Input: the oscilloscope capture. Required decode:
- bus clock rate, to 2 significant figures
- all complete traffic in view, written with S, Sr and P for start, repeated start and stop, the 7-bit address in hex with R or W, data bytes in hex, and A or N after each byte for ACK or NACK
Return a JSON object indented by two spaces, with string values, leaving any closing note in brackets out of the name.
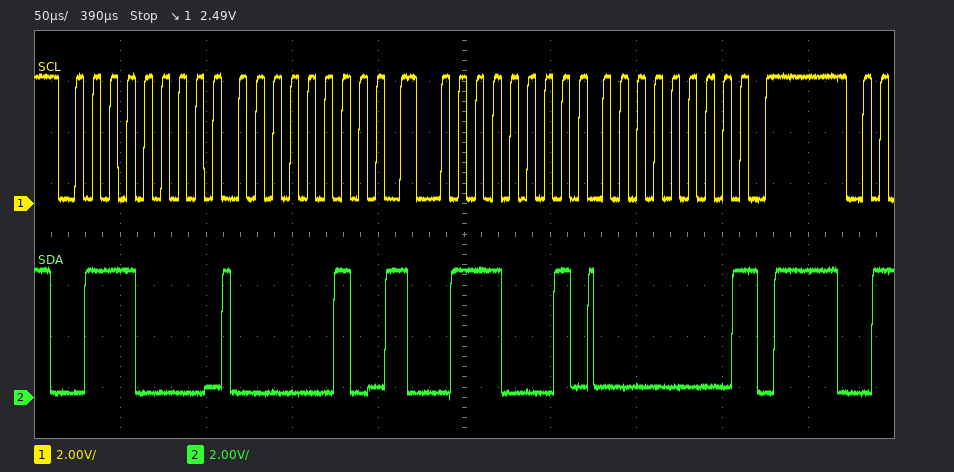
{
  "bus clock rate, to 2 significant figures": "100 kHz",
  "all complete traffic in view, written with S, Sr and P for start, repeated start and stop, the 7-bit address in hex with R or W, data bytes in hex, and A or N after each byte for ACK or NACK": "S 38W A 02 A Sr 38R A 00 N P"
}
